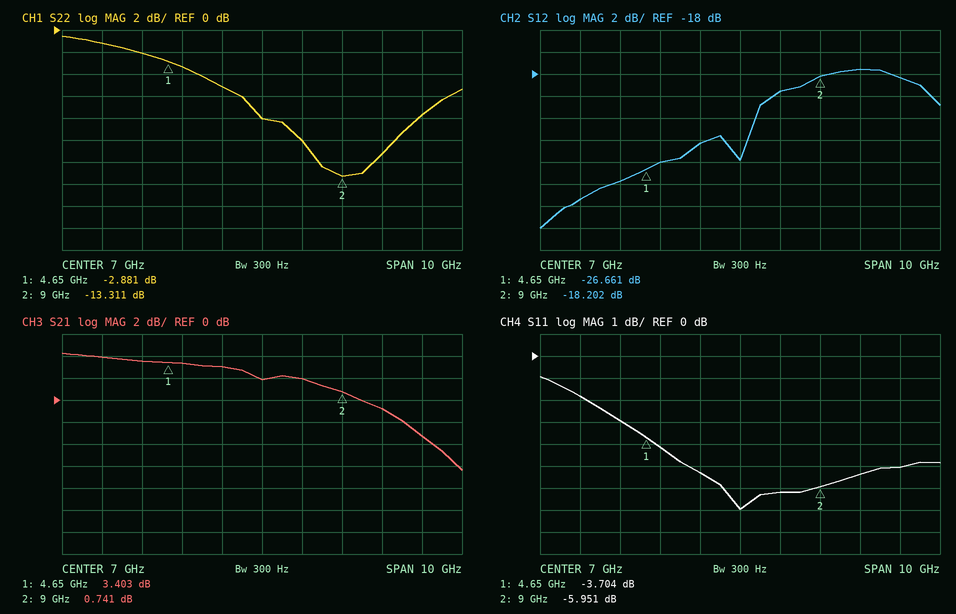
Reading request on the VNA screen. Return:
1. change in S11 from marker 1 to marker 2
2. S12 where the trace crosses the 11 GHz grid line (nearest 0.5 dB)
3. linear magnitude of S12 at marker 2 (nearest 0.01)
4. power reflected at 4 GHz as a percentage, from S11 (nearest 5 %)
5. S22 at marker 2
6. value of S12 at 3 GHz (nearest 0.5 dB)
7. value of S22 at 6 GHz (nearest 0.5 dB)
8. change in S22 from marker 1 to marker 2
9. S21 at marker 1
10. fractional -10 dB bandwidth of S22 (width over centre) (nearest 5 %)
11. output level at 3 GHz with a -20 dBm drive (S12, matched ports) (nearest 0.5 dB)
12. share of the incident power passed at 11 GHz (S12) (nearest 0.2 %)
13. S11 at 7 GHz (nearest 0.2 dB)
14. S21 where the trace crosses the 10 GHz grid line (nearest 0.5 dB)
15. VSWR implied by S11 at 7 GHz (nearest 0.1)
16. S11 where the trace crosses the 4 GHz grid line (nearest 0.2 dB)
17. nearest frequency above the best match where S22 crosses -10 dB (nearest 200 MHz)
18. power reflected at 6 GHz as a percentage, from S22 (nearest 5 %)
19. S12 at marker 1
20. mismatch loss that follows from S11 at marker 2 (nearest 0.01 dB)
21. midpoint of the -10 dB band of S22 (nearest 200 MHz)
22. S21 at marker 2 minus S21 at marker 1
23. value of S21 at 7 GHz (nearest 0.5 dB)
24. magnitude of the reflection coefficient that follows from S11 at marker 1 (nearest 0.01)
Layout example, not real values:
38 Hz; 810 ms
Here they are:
-2.247 dB; -18.5 dB; 0.12; 50 %; -13.311 dB; -29.5 dB; -5.0 dB; -10.430 dB; 3.403 dB; 25 %; -49.5 dBm; 1.4 %; -7.0 dB; -1.0 dB; 2.6; -3.0 dB; 10.4 GHz; 30 %; -26.661 dB; 1.27 dB; 9.2 GHz; -2.662 dB; 2.0 dB; 0.65
